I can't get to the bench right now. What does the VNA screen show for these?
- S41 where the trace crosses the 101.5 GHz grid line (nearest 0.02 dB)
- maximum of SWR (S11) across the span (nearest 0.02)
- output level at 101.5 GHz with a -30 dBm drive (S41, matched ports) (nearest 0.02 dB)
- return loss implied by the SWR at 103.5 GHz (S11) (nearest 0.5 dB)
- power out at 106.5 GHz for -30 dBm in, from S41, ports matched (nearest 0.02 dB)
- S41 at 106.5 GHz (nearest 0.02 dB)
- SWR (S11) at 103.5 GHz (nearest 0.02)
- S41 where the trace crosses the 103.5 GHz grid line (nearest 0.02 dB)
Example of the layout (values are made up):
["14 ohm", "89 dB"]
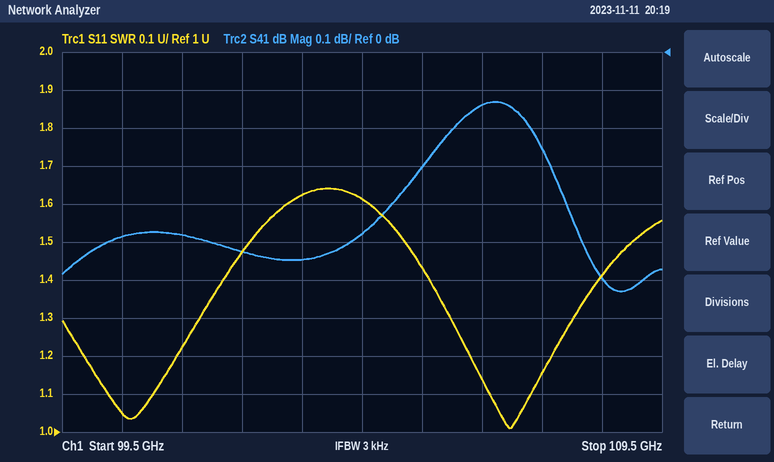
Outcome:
["-0.48 dB", "1.64", "-30.48 dBm", "12.5 dB", "-30.14 dBm", "-0.14 dB", "1.62", "-0.54 dB"]
